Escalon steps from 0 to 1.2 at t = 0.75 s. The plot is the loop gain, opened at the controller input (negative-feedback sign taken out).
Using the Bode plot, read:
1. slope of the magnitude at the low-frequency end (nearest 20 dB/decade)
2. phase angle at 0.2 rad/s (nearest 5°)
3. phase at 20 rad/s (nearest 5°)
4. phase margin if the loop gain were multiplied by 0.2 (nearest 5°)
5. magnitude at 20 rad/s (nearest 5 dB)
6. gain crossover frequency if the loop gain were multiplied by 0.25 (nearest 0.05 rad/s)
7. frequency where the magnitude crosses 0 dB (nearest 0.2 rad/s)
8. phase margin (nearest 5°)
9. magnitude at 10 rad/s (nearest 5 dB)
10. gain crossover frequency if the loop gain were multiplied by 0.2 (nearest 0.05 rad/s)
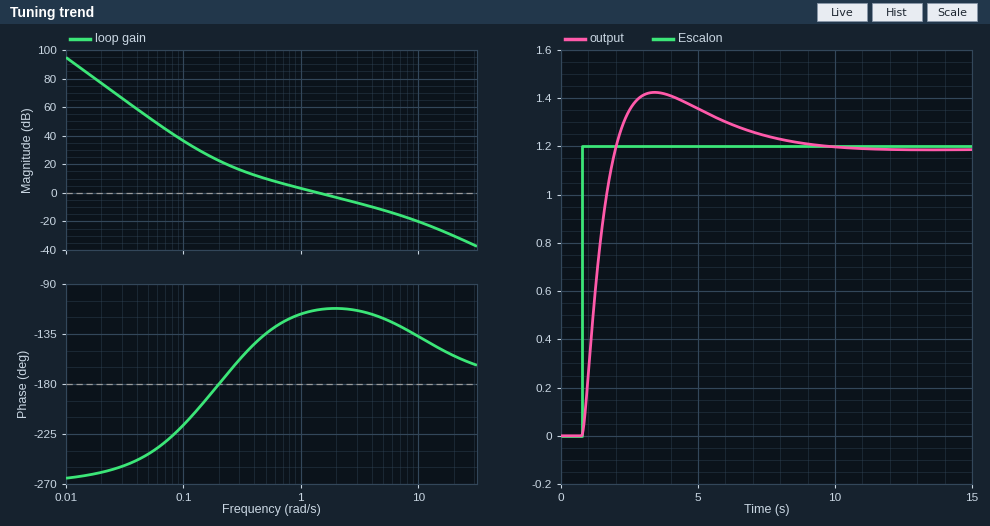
-60 dB/decade
-180°
-155°
30°
-30 dB
0.40 rad/s
1.4 rad/s
65°
-20 dB
0.35 rad/s
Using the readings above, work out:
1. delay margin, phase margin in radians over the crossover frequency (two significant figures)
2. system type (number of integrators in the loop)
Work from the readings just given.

0.81 s
3
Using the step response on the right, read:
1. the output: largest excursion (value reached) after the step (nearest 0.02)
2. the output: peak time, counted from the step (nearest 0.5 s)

1.42
2.5 s
